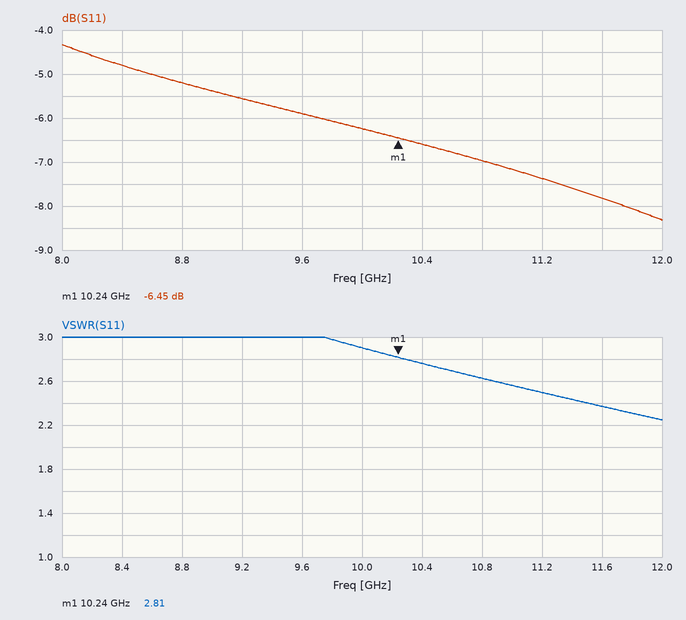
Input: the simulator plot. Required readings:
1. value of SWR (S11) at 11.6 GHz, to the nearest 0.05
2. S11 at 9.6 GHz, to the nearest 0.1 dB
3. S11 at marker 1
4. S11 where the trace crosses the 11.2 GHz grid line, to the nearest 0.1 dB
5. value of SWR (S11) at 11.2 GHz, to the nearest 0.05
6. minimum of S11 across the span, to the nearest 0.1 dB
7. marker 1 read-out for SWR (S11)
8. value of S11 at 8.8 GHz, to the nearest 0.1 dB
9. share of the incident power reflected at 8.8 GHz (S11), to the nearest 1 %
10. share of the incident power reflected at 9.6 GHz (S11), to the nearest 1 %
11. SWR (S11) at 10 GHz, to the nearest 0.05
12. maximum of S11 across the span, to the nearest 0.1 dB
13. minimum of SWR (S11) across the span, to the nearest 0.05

2.35
-5.9 dB
-6.45 dB
-7.4 dB
2.50
-8.3 dB
2.81
-5.2 dB
30 %
26 %
2.90
-4.3 dB
2.25
